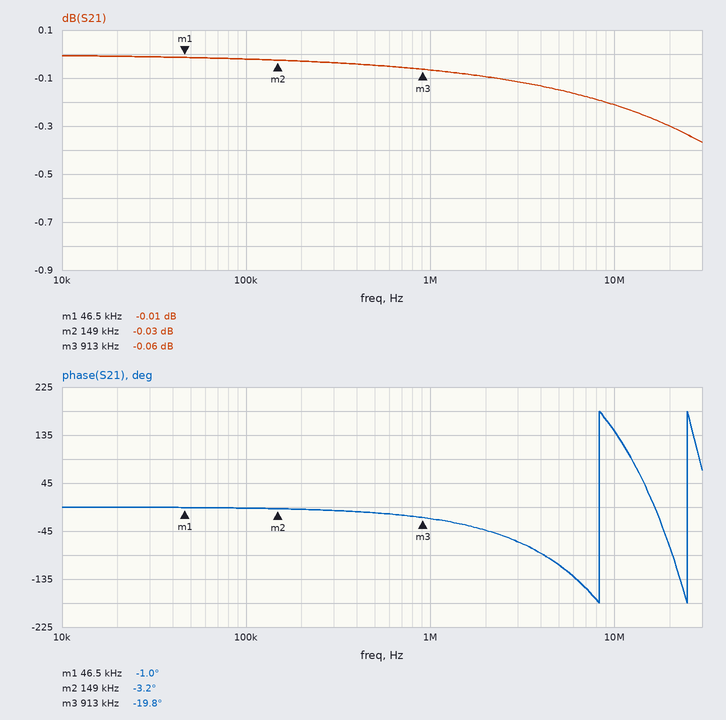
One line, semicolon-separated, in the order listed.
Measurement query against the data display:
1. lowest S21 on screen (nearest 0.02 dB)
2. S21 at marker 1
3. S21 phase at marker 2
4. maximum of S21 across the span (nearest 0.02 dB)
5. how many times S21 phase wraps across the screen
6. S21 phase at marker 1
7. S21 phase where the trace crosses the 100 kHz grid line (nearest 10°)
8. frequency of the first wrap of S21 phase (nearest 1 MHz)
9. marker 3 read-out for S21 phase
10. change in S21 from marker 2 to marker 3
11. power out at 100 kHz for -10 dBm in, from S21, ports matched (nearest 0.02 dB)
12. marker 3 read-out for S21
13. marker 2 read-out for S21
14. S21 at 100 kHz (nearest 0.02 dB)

-0.36 dB; -0.01 dB; -3.2°; 0.00 dB; 2; -1.0°; 0°; 8 MHz; -19.8°; -0.03 dB; -10.02 dBm; -0.06 dB; -0.03 dB; -0.02 dB
